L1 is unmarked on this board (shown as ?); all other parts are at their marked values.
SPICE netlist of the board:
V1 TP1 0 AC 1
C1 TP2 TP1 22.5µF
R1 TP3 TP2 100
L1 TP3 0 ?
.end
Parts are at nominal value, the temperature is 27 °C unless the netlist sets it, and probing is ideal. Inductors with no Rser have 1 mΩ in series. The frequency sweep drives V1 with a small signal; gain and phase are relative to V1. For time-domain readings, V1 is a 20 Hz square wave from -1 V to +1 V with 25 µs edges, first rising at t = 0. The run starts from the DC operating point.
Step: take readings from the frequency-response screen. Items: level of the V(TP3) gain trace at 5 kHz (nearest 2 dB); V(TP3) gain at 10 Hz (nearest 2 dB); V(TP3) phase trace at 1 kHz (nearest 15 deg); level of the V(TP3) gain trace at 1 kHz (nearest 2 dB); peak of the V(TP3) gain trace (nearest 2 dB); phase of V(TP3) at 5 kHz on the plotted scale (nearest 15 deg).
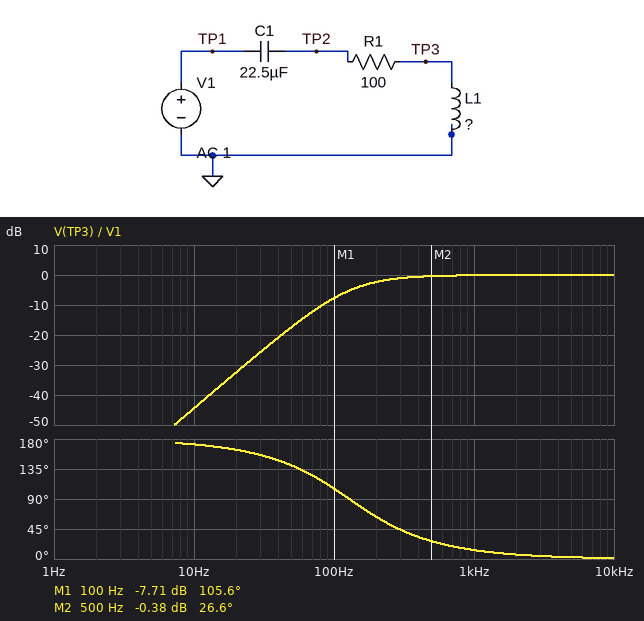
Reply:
0 dB
-44 dB
15 deg
0 dB
0 dB
0 deg
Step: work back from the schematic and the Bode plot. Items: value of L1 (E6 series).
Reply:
68 mH
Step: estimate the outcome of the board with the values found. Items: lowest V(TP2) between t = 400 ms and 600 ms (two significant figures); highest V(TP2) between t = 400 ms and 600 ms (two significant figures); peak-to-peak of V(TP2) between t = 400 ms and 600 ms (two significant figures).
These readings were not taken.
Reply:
-2.0 V
2.0 V
4.0 V
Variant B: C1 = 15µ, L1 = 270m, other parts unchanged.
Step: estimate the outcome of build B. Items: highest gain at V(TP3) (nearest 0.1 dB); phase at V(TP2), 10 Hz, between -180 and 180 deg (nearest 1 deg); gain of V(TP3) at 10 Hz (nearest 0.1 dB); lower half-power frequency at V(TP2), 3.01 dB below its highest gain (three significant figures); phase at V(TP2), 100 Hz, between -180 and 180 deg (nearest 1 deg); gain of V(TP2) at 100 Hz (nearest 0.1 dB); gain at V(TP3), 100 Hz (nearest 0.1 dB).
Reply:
3.2 dB
94 deg
-35.8 dB
62.3 Hz
27 deg
4.4 dB
3.1 dB
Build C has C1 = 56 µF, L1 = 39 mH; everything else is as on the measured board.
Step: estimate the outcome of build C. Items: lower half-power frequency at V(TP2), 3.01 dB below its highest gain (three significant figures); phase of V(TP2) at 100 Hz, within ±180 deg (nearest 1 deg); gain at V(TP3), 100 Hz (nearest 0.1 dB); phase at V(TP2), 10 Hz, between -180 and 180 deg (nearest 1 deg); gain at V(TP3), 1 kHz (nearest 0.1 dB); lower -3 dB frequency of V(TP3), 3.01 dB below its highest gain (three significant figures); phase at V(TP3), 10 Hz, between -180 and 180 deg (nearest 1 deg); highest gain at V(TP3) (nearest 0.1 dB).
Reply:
29.1 Hz
16 deg
-12.2 dB
72 deg
-0.6 dB
380 Hz
160 deg
0 dB
